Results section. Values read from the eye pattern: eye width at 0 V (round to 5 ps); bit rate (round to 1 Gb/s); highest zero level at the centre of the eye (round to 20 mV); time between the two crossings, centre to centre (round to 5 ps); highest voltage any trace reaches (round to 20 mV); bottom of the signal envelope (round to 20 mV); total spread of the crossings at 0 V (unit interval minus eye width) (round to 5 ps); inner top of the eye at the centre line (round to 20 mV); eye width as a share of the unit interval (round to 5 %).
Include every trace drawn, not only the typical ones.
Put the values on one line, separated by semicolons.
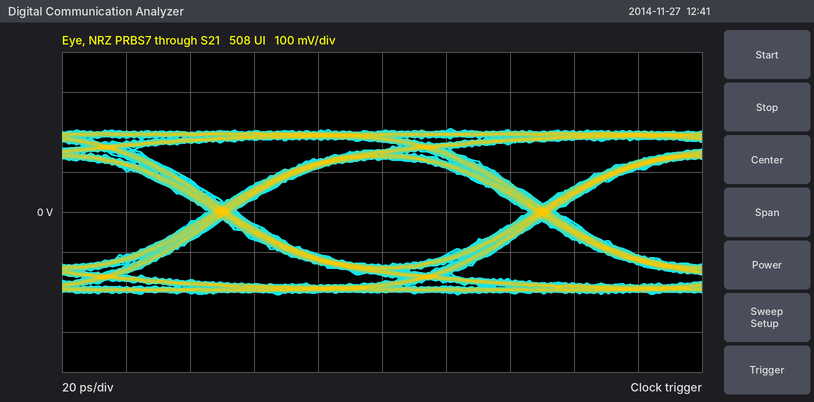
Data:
90 ps; 10 Gb/s; -140 mV; 100 ps; 200 mV; -200 mV; 10 ps; 140 mV; 90 %
